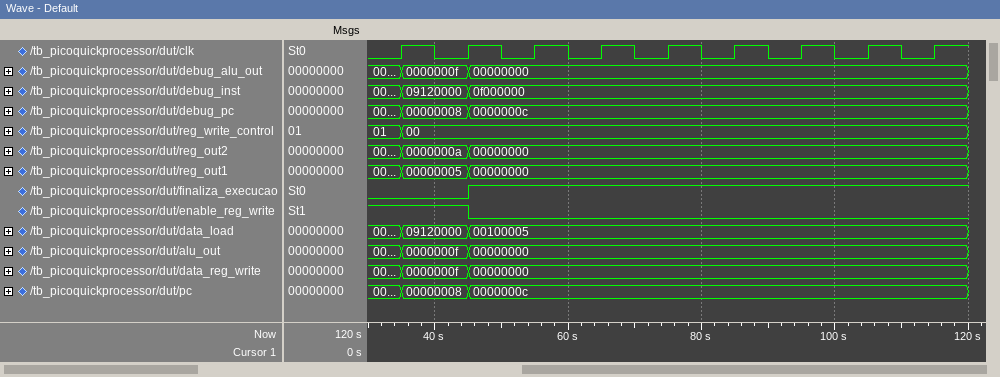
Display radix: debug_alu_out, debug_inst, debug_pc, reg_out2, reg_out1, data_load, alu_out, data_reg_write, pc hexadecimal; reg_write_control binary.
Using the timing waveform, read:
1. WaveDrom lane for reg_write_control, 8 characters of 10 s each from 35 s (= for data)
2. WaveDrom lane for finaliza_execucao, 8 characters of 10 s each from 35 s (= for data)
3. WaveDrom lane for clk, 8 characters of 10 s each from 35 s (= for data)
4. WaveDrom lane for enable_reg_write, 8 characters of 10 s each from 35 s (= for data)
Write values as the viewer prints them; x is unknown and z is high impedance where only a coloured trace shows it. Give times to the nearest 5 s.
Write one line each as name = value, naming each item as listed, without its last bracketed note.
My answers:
WaveDrom lane for reg_write_control, 8 characters of 10 s each from 35 s = {name: 'reg_write_control', wave: '=.......', data: '00'}
WaveDrom lane for finaliza_execucao, 8 characters of 10 s each from 35 s = {name: 'finaliza_execucao', wave: '01......'}
WaveDrom lane for clk, 8 characters of 10 s each from 35 s = {name: 'clk', wave: 'p.......'}
WaveDrom lane for enable_reg_write, 8 characters of 10 s each from 35 s = {name: 'enable_reg_write', wave: '10......'}
